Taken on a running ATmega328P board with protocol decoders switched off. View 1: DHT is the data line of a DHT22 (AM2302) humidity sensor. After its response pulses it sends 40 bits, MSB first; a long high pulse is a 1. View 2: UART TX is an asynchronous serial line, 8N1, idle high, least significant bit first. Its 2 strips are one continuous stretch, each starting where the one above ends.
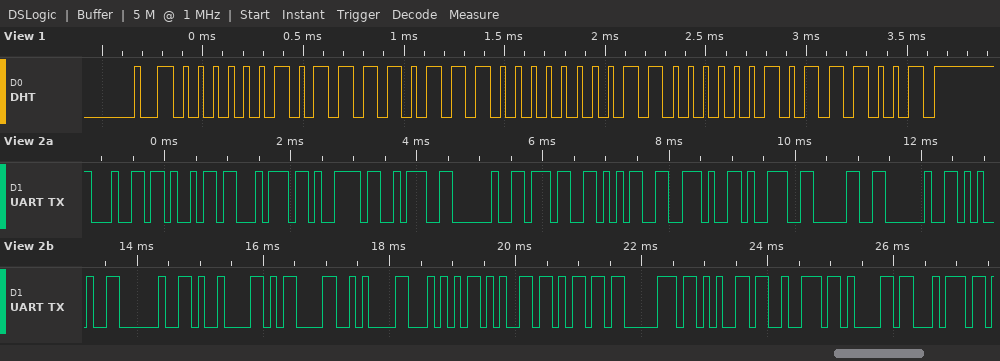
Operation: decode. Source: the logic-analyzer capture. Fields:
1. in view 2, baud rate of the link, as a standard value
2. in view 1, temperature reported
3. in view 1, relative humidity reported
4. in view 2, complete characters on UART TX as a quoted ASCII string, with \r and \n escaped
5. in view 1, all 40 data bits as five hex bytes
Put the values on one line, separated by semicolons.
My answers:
9600 baud; 19.2 °C; 75.9 %; "dity: 75.90 % \t\r\nTemperat"; 02 F7 00 C0 B9
